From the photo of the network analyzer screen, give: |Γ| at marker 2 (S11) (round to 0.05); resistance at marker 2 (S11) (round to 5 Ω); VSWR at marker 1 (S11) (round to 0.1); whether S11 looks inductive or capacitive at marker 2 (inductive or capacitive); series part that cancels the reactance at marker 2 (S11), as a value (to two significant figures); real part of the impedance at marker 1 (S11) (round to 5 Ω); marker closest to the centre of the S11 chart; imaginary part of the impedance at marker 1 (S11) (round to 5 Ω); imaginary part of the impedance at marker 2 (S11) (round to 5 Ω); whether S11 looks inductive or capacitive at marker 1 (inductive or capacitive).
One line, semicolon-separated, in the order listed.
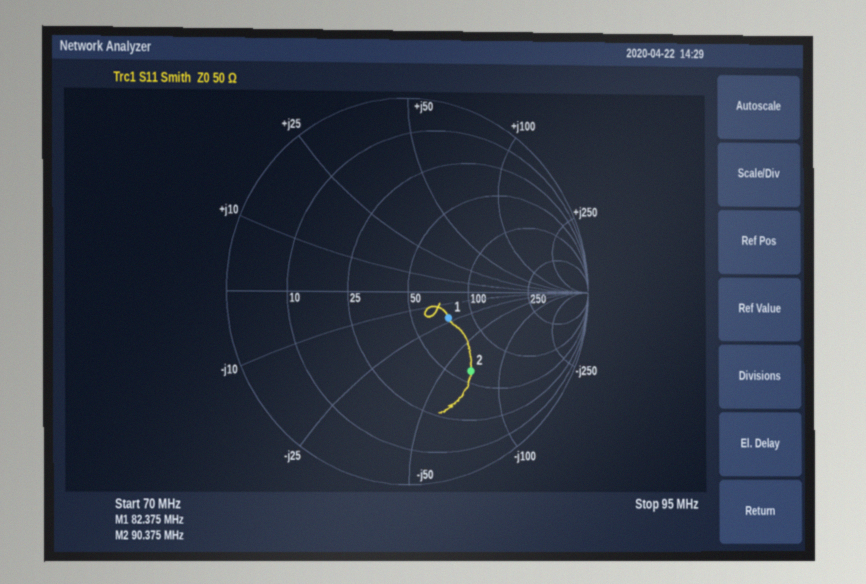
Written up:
0.55; 60 Ω; 1.7; capacitive; 120 nH; 75 Ω; marker 1; -20 Ω; -70 Ω; capacitive
